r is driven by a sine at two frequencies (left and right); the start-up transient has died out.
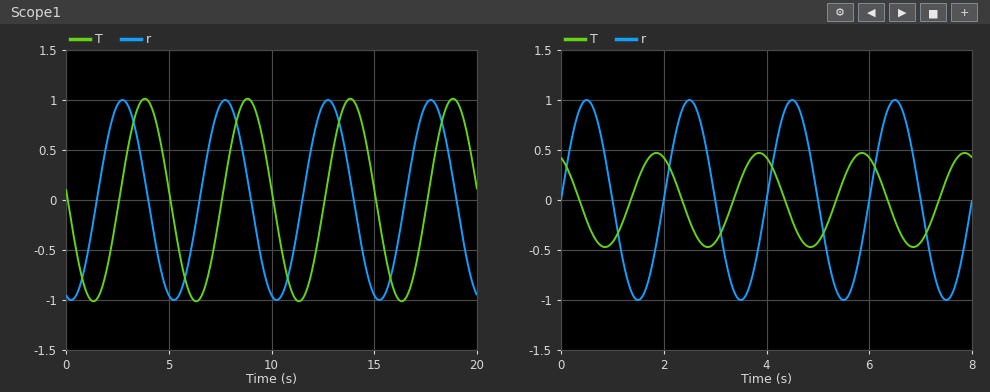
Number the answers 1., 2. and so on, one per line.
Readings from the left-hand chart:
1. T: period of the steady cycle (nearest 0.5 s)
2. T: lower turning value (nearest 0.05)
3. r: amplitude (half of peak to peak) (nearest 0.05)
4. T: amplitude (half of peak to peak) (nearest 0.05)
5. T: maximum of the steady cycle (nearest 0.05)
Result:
1. 5.0 s
2. -1.00
3. 1.00
4. 1.00
5. 1.00
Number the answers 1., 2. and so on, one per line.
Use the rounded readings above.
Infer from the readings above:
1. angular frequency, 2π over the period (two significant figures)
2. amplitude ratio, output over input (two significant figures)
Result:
1. 1.3 rad/s
2. 1.0
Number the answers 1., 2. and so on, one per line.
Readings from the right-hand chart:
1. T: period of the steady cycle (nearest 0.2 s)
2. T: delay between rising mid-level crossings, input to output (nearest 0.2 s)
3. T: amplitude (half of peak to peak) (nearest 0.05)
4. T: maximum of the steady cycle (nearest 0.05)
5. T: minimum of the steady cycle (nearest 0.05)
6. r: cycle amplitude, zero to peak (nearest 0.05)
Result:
1. 2.0 s
2. 1.4 s
3. 0.45
4. 0.45
5. -0.45
6. 1.00
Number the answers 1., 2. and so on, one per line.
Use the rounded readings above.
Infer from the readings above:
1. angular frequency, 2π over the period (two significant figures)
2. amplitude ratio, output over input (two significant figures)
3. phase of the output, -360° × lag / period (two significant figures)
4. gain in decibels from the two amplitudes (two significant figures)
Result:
1. 3.1 rad/s
2. 0.45
3. -250°
4. -6.9 dB
